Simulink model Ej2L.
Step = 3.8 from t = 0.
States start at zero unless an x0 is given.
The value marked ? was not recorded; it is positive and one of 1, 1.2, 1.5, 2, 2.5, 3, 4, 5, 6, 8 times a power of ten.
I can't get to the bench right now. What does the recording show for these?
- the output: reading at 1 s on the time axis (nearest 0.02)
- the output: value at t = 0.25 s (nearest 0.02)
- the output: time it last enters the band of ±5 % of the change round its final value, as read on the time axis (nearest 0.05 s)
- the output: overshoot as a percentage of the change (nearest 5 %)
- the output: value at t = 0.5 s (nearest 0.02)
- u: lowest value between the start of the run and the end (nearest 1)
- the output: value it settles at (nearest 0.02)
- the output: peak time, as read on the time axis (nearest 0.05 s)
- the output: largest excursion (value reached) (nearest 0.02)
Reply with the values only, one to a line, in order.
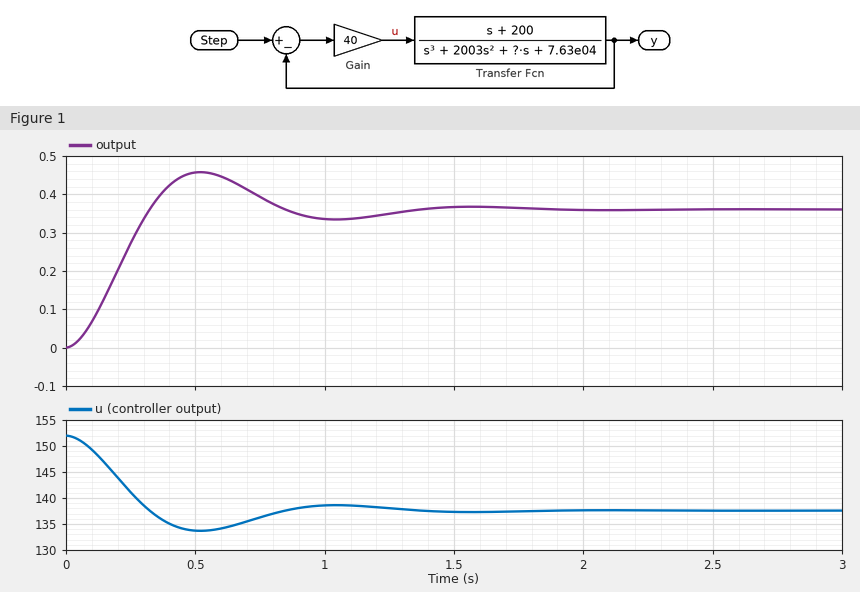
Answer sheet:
0.34
0.28
1.20 s
25 %
0.46
134
0.36
0.50 s
0.46
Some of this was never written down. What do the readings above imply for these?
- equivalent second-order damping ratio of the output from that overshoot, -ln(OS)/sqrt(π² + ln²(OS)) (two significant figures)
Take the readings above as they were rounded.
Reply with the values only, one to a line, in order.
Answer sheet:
0.40
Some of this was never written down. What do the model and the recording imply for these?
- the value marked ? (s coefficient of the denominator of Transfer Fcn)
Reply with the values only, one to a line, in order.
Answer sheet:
10000
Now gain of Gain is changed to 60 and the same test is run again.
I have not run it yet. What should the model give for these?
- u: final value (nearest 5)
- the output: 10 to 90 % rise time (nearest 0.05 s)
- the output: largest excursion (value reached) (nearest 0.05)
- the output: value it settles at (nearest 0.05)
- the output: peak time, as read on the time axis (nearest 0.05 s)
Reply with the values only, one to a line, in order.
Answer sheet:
195
0.20 s
0.65
0.50
0.50 s
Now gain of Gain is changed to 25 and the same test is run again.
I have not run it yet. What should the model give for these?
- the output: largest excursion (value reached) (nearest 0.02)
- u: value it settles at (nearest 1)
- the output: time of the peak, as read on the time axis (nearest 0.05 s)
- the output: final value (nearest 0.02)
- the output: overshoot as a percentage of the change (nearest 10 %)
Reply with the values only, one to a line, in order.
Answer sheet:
0.30
89
0.55 s
0.24
30 %
